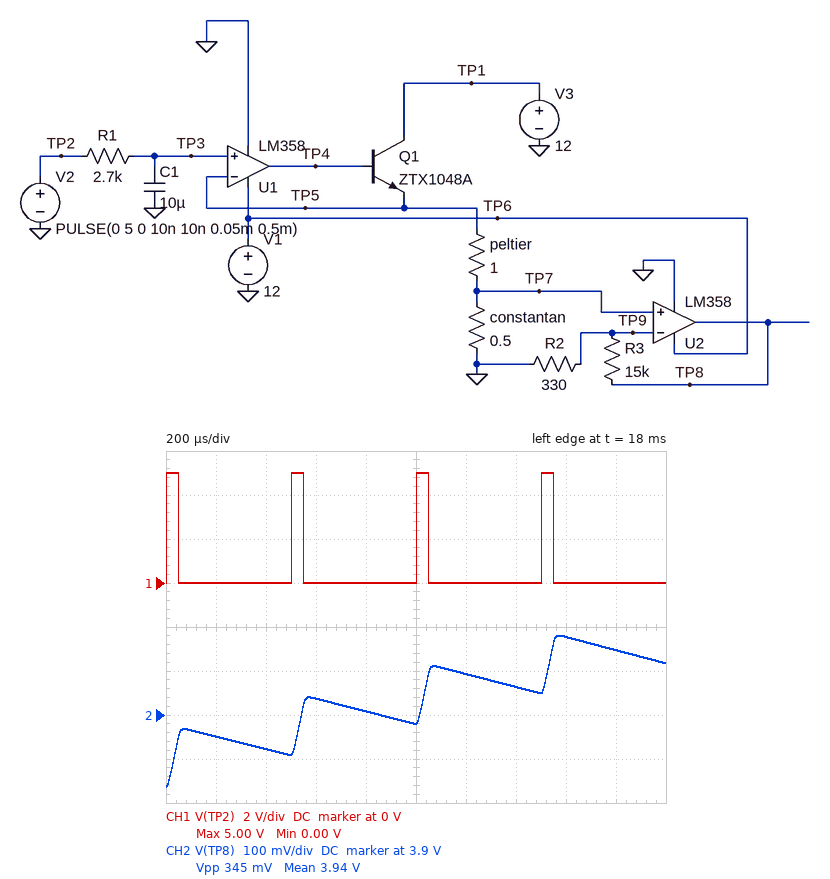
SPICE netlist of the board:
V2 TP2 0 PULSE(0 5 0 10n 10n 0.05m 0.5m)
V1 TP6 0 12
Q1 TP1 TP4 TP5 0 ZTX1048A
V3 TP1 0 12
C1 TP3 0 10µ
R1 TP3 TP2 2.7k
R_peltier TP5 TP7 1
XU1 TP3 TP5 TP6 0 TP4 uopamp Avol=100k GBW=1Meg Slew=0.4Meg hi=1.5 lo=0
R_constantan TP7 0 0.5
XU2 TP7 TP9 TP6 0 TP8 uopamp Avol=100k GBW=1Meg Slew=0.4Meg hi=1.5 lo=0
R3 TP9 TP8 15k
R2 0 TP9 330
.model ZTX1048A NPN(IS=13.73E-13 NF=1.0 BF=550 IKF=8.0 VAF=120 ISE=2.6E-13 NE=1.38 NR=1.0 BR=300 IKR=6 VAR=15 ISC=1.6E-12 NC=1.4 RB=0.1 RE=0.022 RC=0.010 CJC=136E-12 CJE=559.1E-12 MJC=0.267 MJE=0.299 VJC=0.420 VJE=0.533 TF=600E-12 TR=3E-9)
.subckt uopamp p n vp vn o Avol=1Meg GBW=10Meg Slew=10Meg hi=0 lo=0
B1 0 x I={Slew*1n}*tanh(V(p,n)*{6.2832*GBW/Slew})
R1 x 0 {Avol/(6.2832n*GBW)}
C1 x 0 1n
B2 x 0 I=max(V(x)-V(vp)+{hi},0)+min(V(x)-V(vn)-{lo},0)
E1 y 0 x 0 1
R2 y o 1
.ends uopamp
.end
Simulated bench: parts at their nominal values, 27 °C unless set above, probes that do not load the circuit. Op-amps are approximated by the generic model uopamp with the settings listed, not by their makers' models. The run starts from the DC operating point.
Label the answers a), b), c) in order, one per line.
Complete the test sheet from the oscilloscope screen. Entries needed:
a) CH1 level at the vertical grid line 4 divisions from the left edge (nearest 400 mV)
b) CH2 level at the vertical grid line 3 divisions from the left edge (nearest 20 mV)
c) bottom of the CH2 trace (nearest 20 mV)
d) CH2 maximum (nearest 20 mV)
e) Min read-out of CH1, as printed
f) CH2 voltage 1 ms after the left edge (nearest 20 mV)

a) 0 V
b) 3.94 V
c) 3.74 V
d) 4.08 V
e) 0.00 V
f) 3.88 V
